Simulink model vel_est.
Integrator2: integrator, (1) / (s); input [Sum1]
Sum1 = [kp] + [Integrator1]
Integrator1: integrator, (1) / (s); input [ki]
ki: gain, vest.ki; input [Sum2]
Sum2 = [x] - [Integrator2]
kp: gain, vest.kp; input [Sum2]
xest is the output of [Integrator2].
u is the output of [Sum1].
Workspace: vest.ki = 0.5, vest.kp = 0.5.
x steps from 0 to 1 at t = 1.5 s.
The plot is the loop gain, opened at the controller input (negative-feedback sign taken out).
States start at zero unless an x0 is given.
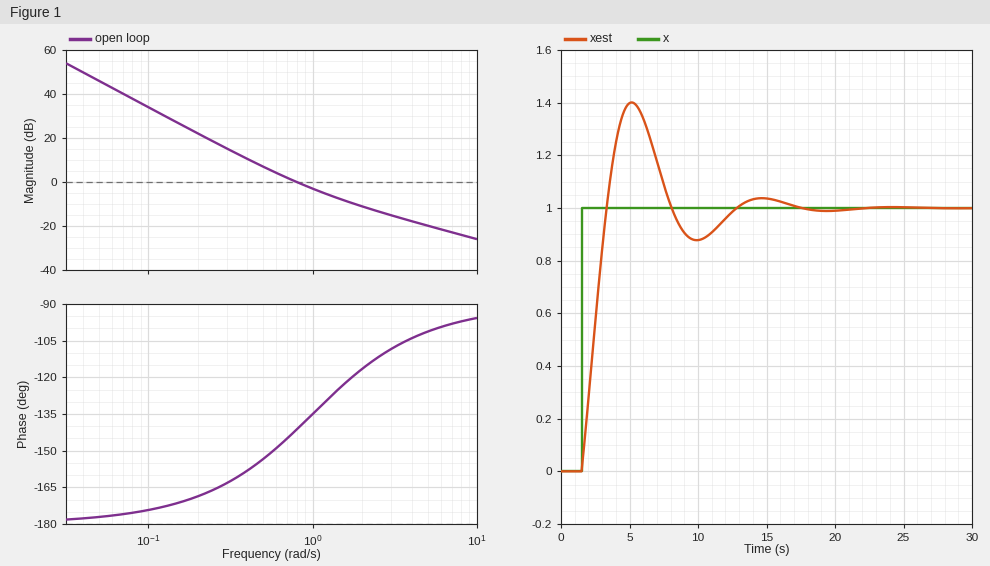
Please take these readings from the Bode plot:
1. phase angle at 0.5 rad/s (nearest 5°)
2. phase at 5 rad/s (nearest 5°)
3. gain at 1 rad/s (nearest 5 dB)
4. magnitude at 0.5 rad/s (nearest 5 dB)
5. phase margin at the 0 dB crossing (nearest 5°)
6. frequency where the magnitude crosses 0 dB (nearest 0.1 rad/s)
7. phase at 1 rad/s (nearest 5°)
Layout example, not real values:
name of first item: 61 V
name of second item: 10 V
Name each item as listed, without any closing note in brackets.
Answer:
phase angle at 0.5 rad/s: -155°
phase at 5 rad/s: -100°
gain at 1 rad/s: -5 dB
magnitude at 0.5 rad/s: 5 dB
phase margin at the 0 dB crossing: 40°
frequency where the magnitude crosses 0 dB: 0.8 rad/s
phase at 1 rad/s: -135°
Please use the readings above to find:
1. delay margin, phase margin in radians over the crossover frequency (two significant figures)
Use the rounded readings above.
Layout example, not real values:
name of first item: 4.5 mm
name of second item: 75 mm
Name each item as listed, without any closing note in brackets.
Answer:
delay margin, phase margin in radians over the crossover frequency: 0.87 s
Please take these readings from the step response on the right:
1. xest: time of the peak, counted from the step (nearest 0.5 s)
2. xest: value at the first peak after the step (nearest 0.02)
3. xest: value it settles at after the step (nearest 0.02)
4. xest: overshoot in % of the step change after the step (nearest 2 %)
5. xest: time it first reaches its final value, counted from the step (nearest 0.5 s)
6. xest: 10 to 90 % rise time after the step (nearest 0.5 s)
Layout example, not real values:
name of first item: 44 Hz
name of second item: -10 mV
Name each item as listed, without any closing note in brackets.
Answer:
xest: time of the peak, counted from the step: 3.5 s
xest: value at the first peak after the step: 1.40
xest: value it settles at after the step: 1.00
xest: overshoot in % of the step change after the step: 40 %
xest: time it first reaches its final value, counted from the step: 2.0 s
xest: 10 to 90 % rise time after the step: 1.5 s
